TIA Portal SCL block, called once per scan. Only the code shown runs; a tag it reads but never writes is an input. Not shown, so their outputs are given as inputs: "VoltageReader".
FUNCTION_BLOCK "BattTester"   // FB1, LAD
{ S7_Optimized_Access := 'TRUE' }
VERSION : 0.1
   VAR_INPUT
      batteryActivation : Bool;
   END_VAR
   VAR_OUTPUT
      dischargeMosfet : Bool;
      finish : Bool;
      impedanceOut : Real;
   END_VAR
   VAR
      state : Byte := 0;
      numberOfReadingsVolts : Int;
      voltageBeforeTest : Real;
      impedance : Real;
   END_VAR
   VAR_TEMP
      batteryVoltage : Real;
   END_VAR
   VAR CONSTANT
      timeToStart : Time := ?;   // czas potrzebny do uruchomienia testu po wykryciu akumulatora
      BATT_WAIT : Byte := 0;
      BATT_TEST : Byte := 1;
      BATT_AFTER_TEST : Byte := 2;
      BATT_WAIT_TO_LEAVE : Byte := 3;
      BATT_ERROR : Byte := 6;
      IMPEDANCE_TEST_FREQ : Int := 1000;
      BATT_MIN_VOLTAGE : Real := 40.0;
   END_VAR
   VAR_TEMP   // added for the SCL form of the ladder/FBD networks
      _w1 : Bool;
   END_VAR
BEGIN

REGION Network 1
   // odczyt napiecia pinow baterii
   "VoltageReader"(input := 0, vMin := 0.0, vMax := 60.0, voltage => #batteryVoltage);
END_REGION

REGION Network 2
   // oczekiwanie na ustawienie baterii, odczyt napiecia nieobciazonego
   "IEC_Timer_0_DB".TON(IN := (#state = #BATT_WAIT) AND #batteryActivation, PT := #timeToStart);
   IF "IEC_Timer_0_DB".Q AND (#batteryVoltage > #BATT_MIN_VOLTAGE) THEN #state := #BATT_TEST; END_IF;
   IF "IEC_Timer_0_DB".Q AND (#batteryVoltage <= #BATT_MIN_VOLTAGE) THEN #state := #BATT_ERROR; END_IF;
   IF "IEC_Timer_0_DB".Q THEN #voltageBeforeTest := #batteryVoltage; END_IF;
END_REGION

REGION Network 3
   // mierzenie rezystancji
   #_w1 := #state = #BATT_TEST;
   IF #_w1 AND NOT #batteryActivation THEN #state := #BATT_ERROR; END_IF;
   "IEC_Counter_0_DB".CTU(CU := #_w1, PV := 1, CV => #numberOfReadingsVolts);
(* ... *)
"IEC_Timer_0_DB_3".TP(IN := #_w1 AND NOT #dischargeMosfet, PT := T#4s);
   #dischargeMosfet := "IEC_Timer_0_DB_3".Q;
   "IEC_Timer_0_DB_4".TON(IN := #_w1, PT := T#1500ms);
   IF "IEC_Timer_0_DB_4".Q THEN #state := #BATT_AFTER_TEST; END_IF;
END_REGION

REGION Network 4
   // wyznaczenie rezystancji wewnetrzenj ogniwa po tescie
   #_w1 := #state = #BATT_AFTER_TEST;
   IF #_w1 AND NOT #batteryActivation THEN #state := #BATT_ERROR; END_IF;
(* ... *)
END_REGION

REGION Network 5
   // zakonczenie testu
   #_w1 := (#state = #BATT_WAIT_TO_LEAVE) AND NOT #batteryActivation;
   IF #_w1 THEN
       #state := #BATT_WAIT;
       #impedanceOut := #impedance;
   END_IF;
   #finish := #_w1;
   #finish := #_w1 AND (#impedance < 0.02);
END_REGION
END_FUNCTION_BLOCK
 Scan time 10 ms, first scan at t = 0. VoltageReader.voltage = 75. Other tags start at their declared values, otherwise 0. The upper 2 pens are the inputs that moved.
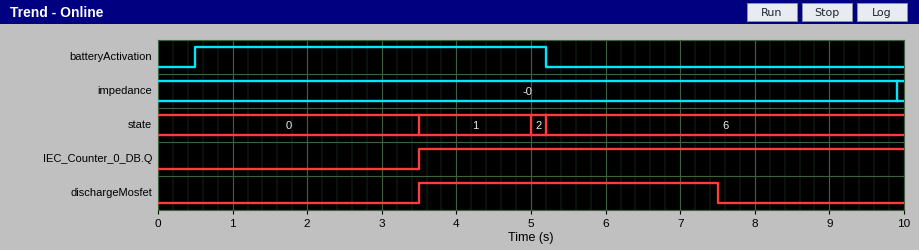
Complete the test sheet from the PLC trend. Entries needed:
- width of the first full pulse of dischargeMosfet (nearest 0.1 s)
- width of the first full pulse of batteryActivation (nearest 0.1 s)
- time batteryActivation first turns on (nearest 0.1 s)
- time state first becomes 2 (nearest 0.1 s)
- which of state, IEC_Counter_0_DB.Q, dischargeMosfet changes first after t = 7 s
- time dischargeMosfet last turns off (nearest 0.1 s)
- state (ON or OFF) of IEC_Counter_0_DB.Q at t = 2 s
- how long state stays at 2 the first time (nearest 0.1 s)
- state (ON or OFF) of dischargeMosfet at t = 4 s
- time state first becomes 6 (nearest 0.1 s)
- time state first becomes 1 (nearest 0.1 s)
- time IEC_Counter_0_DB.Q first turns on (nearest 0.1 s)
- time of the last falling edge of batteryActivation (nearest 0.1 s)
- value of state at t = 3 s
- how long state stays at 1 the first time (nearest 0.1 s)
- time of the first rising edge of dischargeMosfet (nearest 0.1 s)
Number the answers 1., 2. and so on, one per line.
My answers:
1. 4.0 s
2. 4.7 s
3. 0.5 s
4. 5.0 s
5. dischargeMosfet
6. 7.5 s
7. OFF
8. 0.2 s
9. ON
10. 5.2 s
11. 3.5 s
12. 3.5 s
13. 5.2 s
14. 0
15. 1.5 s
16. 3.5 s
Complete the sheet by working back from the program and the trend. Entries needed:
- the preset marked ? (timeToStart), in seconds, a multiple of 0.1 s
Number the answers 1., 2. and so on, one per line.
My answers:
1. 3.0 s
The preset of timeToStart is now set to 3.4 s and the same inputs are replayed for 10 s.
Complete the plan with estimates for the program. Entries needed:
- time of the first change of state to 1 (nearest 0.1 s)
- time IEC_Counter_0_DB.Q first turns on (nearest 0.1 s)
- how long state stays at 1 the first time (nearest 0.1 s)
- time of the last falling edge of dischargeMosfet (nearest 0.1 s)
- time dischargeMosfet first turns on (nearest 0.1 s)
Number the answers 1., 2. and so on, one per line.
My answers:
1. 3.9 s
2. 3.9 s
3. 1.3 s
4. 7.9 s
5. 3.9 s
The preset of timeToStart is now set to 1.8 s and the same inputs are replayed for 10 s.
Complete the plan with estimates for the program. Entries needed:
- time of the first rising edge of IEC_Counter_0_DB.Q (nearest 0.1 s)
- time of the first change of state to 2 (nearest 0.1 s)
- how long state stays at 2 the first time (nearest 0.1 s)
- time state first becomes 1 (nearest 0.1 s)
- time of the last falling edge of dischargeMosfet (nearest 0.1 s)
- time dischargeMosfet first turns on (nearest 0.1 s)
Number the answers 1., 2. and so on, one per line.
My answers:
1. 2.3 s
2. 3.8 s
3. 1.4 s
4. 2.3 s
5. 6.3 s
6. 2.3 s
